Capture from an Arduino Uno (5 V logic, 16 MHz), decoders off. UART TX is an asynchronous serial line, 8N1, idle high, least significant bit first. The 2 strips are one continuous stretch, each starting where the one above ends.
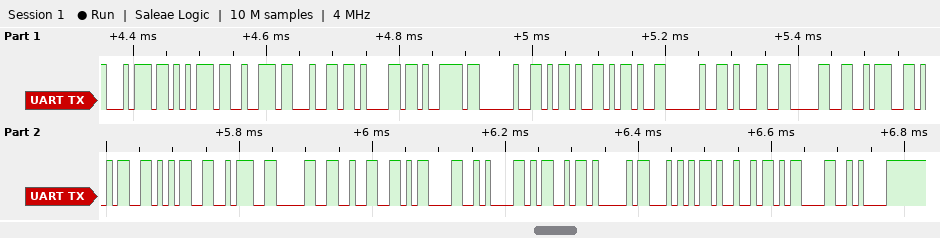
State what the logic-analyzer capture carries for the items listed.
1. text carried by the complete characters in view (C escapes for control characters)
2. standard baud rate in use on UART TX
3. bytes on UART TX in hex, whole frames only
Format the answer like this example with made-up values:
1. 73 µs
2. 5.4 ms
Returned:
1. "turday -- 10:55:02\r\nMATI\r\n"
2. 115200 baud
3. 74 75 72 64 61 79 20 2D 2D 20 31 30 3A 35 35 3A 30 32 0D 0A 4D 41 54 49 0D 0A
